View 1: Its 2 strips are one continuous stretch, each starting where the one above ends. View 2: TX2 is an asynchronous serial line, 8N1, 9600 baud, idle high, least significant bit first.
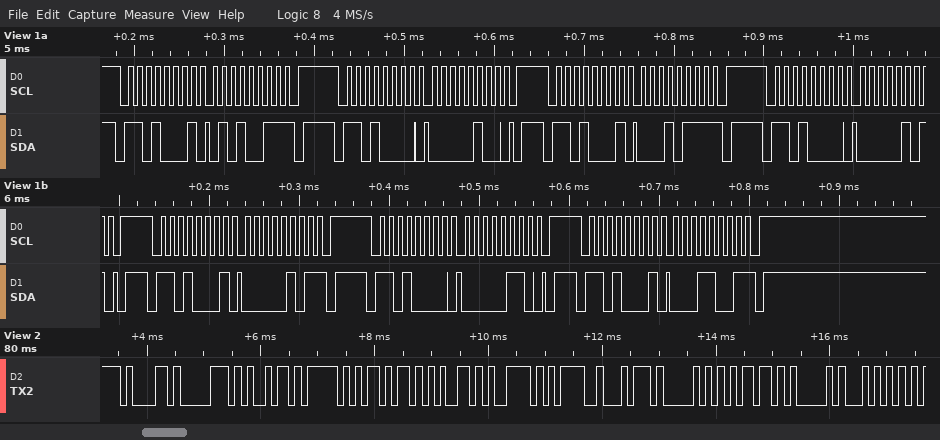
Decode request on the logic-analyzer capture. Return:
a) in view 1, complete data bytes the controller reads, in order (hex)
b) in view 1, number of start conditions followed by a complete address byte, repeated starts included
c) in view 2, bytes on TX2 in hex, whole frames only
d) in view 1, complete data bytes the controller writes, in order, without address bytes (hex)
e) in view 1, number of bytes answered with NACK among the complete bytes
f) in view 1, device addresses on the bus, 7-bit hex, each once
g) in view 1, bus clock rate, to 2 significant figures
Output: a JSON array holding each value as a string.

["53 17 05 19", "7", "0x61 0x70 0x69 0x5F 0x6B 0x65 0x79 0x3D 0x74 0x50 0x6D 0x41 0x54", "04 05 06", "4", "0x68", "100 kHz"]
